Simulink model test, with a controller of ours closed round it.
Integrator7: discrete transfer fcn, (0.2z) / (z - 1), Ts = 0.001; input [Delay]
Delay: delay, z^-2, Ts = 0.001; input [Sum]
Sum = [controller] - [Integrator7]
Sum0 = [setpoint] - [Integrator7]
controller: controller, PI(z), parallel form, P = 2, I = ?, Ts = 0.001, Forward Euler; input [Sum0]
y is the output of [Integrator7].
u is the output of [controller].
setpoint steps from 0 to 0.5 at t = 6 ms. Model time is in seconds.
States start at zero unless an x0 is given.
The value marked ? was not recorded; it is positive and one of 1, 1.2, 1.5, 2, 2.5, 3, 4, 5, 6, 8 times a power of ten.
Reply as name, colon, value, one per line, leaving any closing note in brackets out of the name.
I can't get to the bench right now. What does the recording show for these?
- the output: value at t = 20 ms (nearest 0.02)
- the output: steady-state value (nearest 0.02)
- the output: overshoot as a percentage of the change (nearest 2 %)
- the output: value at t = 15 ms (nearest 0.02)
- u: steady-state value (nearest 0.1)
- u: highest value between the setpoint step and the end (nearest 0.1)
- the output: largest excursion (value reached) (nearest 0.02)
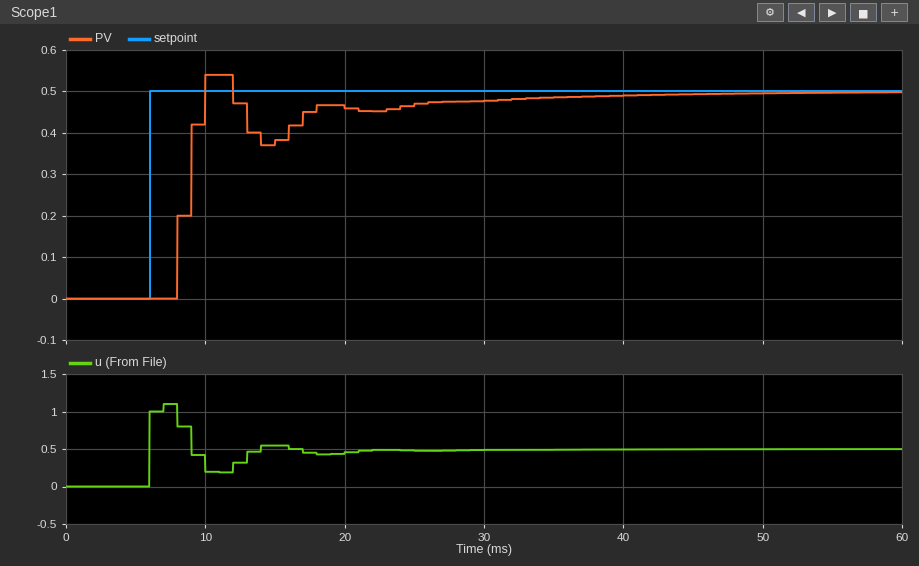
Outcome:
the output: value at t = 20 ms: 0.46
the output: steady-state value: 0.50
the output: overshoot as a percentage of the change: 8 %
the output: value at t = 15 ms: 0.38
u: steady-state value: 0.5
u: highest value between the setpoint step and the end: 1.1
the output: largest excursion (value reached): 0.54
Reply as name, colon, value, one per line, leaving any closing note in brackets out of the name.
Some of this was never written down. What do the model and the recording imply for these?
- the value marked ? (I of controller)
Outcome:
the value marked ?: 200
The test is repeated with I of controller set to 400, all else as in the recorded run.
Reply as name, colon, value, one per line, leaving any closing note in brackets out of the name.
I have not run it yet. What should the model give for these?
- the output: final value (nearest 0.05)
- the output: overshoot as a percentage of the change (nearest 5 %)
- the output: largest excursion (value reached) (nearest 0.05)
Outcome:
the output: final value: 0.50
the output: overshoot as a percentage of the change: 30 %
the output: largest excursion (value reached): 0.65
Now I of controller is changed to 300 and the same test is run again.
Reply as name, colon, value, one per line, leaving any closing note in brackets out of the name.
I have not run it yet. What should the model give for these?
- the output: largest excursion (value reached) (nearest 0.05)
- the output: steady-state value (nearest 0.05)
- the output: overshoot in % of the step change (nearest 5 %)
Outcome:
the output: largest excursion (value reached): 0.60
the output: steady-state value: 0.50
the output: overshoot in % of the step change: 20 %
